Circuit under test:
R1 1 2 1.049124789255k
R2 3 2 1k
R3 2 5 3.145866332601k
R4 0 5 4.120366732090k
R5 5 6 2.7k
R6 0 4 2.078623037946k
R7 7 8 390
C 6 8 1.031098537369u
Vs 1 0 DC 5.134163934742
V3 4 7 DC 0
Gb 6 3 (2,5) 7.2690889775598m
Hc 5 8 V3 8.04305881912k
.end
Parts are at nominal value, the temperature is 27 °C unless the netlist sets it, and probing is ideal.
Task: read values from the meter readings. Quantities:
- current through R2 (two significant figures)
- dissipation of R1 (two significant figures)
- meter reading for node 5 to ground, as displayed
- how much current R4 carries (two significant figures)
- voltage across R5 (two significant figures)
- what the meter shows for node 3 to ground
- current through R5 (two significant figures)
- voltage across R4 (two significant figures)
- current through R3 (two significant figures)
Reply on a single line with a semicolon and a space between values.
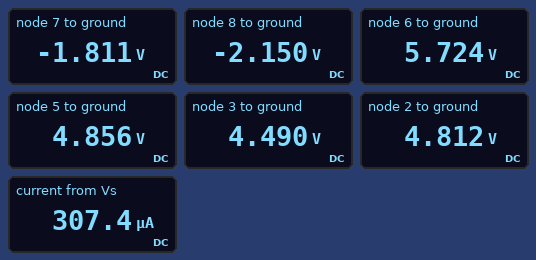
320 µA; 99 µW; 4.856 V; 1.2 mA; 870 mV; 4.490 V; 320 µA; 4.9 V; 14 µA
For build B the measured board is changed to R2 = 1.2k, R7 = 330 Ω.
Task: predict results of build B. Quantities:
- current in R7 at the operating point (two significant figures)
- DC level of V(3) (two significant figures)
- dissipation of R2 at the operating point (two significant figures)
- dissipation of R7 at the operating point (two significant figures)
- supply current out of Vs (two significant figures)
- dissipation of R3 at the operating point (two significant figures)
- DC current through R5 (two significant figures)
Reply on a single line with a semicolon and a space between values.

860 µA; 4.4 V; 130 µW; 240 µW; 320 µA; 660 nW; 330 µA
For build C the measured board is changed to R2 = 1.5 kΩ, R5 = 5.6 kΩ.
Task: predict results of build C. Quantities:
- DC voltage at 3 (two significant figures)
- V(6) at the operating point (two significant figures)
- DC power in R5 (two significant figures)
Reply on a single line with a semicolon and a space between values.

4.3 V; 6.7 V; 580 µW
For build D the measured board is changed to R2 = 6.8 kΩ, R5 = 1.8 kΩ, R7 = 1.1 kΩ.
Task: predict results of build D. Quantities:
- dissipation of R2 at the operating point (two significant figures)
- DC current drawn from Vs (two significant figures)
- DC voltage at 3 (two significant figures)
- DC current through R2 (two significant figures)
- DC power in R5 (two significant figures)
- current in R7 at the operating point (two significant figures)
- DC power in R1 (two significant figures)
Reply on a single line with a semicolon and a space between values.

250 µW; 180 µA; 3.6 V; 190 µA; 67 µW; 1.0 mA; 36 µW
